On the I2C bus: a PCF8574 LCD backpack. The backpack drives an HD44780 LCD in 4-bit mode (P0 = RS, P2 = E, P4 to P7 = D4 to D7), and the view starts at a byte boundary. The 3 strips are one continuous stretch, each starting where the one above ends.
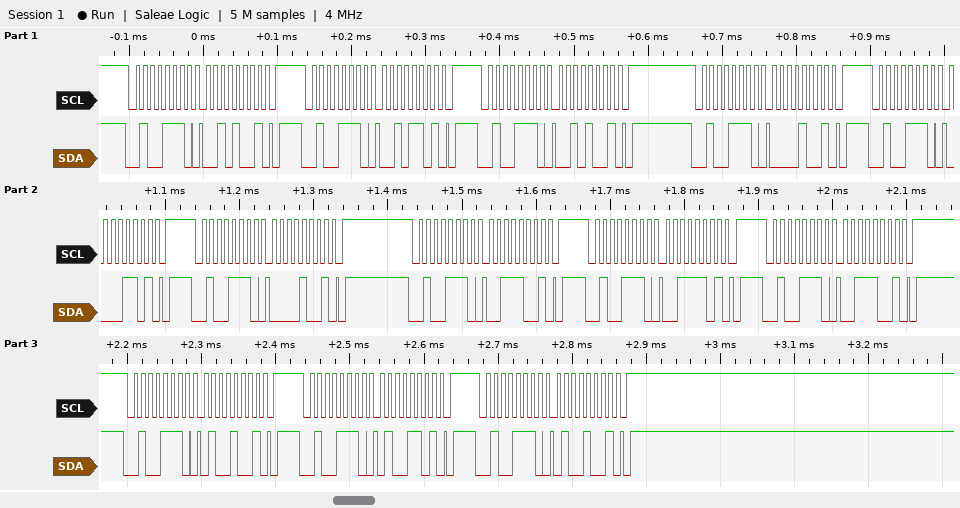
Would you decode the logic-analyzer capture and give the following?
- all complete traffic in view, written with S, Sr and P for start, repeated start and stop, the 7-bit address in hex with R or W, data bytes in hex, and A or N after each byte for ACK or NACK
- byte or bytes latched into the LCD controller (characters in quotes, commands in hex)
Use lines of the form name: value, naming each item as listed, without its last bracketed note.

all complete traffic in view, written with S, Sr and P for start, repeated start and stop, the 7-bit address in hex with R or W, data bytes in hex, and A or N after each byte for ACK or NACK: S 27W A 29 A P S 27W A 2D A P S 27W A 29 A P S 27W A 09 A P S 27W A 0D A P S 27W A 09 A P S 27W A 39 A P S 27W A 3D A P S 27W A 39 A P S 27W A 49 A P S 27W A 4D A P S 27W A 49 A P
byte or bytes latched into the LCD controller: ' ' '4'
